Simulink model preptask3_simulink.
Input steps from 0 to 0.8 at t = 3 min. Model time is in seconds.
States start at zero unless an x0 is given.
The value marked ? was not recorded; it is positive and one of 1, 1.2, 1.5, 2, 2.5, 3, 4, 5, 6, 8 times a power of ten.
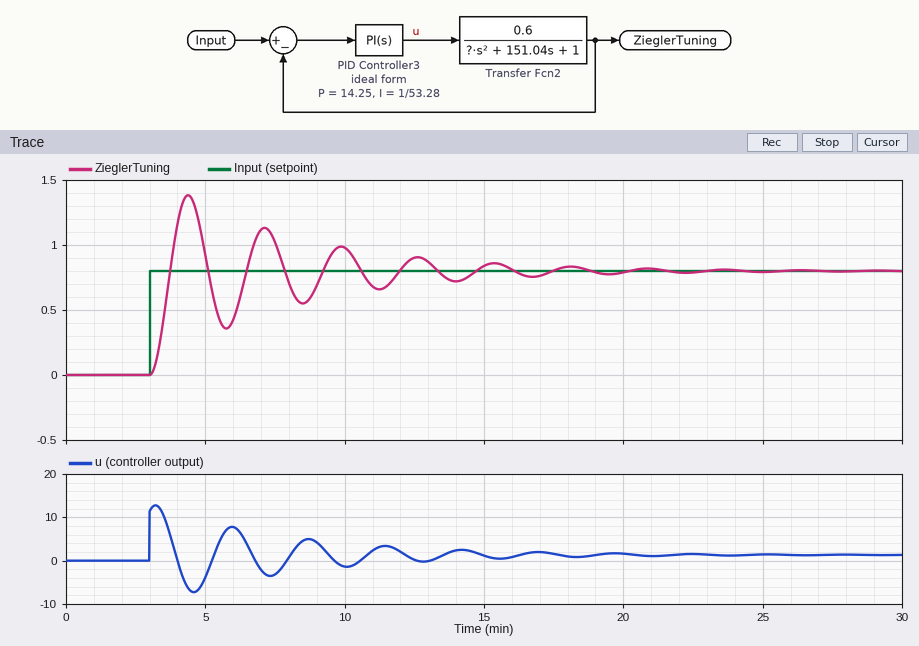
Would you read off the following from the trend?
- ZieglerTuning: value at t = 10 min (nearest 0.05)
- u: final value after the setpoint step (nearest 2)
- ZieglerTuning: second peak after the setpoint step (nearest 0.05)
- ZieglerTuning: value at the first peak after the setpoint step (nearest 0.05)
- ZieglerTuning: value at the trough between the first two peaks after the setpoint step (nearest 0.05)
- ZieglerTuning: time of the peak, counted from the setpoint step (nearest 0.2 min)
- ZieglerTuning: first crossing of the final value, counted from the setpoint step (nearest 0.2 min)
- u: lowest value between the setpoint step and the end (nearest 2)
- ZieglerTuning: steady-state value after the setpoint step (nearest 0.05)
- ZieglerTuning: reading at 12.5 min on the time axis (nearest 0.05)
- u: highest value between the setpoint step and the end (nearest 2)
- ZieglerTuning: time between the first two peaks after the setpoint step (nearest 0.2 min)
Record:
1.00
2
1.15
1.40
0.35
1.4 min
0.8 min
-8
0.80
0.90
12
2.8 min
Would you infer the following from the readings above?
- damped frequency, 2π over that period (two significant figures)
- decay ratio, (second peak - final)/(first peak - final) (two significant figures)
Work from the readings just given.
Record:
2.2 rad/min
0.58
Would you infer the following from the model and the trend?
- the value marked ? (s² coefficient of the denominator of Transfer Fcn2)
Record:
6000
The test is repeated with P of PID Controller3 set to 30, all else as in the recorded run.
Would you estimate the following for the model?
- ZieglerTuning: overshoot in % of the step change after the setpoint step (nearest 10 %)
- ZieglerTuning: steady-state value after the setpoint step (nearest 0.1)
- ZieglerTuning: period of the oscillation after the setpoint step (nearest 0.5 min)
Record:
80 %
0.8
2.0 min
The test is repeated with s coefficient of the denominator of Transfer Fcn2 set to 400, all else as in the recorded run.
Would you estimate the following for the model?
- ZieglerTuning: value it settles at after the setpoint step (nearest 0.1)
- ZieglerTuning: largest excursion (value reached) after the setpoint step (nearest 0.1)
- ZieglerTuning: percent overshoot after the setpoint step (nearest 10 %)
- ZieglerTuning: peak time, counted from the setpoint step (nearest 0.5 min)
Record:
0.8
1.1
40 %
2.0 min
